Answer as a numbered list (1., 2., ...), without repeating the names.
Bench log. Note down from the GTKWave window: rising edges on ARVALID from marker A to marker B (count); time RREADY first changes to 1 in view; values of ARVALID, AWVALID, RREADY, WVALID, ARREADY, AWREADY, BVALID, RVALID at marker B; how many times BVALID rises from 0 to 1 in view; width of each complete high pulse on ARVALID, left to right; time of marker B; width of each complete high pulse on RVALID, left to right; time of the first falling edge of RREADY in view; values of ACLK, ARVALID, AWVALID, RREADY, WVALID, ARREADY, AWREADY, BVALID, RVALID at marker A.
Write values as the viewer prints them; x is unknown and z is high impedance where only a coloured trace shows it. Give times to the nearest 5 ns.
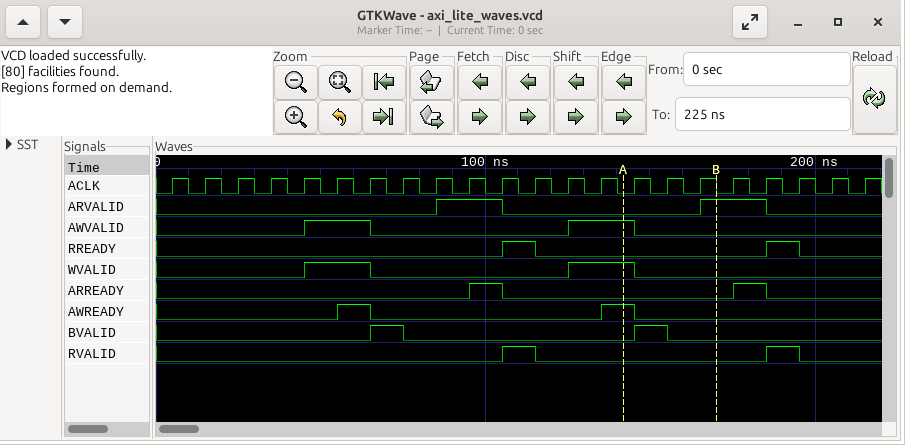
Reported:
1. 1
2. 105 ns
3. ARVALID=1, AWVALID=0, RREADY=0, WVALID=0, ARREADY=0, AWREADY=0, BVALID=0, RVALID=0
4. 2
5. 20 ns, 20 ns
6. 170 ns
7. 10 ns, 10 ns
8. 115 ns
9. ACLK=0, ARVALID=0, AWVALID=1, RREADY=0, WVALID=1, ARREADY=0, AWREADY=1, BVALID=0, RVALID=0
